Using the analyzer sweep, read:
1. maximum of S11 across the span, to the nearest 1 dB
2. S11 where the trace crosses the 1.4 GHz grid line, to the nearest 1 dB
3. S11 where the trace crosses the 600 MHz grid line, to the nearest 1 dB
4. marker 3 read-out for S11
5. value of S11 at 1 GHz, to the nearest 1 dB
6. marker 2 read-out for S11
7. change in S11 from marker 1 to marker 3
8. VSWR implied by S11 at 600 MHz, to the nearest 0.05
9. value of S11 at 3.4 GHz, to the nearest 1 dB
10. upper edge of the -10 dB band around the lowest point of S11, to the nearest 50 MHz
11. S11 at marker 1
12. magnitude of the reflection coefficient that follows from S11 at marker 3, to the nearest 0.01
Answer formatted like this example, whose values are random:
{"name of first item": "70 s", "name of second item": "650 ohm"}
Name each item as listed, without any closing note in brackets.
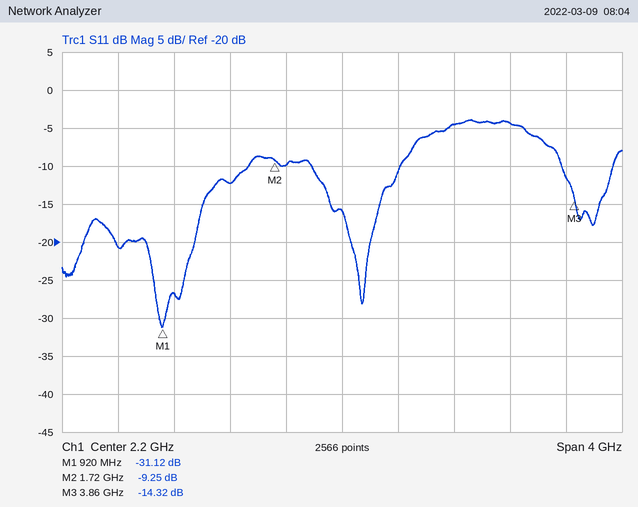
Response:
{"maximum of S11 across the span, to the nearest 1 dB": "-4 dB", "S11 where the trace crosses the 1.4 GHz grid line, to the nearest 1 dB": "-12 dB", "S11 where the trace crosses the 600 MHz grid line, to the nearest 1 dB": "-21 dB", "marker 3 read-out for S11": "-14.32 dB", "value of S11 at 1 GHz, to the nearest 1 dB": "-27 dB", "marker 2 read-out for S11": "-9.25 dB", "change in S11 from marker 1 to marker 3": "16.80 dB", "VSWR implied by S11 at 600 MHz, to the nearest 0.05": "1.20", "value of S11 at 3.4 GHz, to the nearest 1 dB": "-4 dB", "upper edge of the -10 dB band around the lowest point of S11, to the nearest 50 MHz": "1.55 GHz", "S11 at marker 1": "-31.12 dB", "magnitude of the reflection coefficient that follows from S11 at marker 3, to the nearest 0.01": "0.19"}
